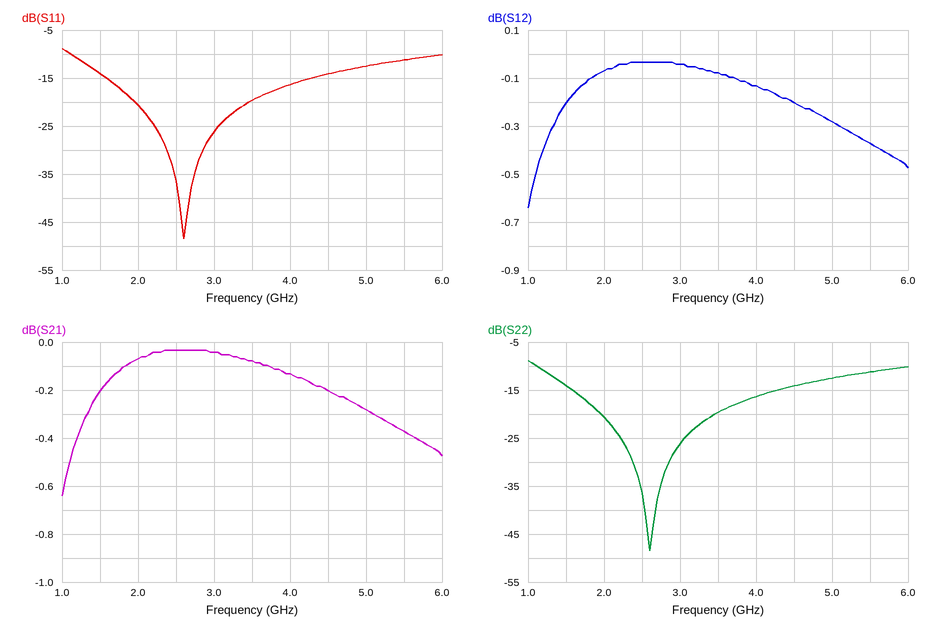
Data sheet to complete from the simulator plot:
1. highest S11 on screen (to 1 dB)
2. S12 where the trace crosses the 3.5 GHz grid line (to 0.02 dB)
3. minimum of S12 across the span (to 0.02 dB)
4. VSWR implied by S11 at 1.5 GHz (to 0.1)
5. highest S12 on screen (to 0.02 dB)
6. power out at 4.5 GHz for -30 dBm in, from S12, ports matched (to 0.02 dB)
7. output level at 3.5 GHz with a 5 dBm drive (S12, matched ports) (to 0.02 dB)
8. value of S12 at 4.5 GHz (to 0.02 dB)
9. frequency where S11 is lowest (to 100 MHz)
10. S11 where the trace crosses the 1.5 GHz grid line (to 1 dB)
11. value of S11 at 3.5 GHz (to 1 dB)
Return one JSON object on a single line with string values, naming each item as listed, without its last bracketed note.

{"highest S11 on screen": "-9 dB", "S12 where the trace crosses the 3.5 GHz grid line": "-0.08 dB", "minimum of S12 across the span": "-0.64 dB", "VSWR implied by S11 at 1.5 GHz": "1.5", "highest S12 on screen": "-0.04 dB", "power out at 4.5 GHz for -30 dBm in, from S12, ports matched": "-30.20 dBm", "output level at 3.5 GHz with a 5 dBm drive (S12, matched ports)": "4.92 dBm", "value of S12 at 4.5 GHz": "-0.20 dB", "frequency where S11 is lowest": "2.6 GHz", "S11 where the trace crosses the 1.5 GHz grid line": "-14 dB", "value of S11 at 3.5 GHz": "-20 dB"}
